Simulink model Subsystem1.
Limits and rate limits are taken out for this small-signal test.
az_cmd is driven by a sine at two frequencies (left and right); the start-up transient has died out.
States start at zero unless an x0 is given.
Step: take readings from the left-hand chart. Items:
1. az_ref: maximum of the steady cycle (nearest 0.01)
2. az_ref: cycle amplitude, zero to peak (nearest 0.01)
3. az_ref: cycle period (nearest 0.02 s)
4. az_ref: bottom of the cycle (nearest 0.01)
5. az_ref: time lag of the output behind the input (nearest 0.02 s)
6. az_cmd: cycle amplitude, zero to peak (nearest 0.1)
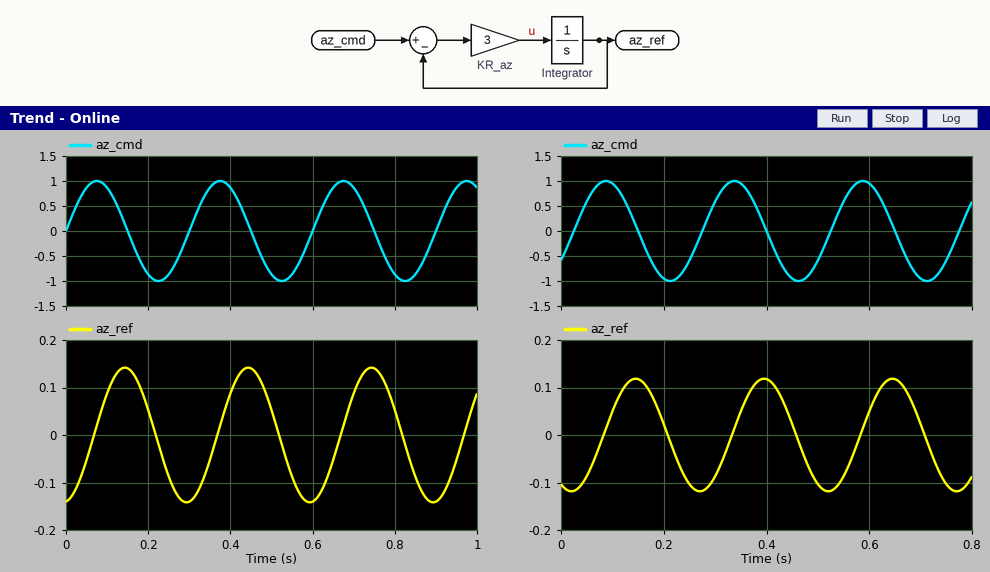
0.14
0.14
0.30 s
-0.14
0.06 s
1.0
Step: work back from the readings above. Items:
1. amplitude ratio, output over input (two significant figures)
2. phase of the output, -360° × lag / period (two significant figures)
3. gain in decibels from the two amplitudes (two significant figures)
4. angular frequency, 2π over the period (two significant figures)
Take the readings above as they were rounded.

0.14
-72°
-17 dB
21 rad/s
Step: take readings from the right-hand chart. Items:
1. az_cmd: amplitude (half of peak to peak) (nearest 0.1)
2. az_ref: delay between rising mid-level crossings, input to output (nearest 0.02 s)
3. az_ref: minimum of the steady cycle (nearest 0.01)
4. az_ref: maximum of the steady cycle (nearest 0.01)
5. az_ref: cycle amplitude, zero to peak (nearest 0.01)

1.0
0.06 s
-0.12
0.12
0.12
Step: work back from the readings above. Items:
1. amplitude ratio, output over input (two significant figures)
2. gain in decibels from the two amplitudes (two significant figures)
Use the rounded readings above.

0.12
-18 dB
